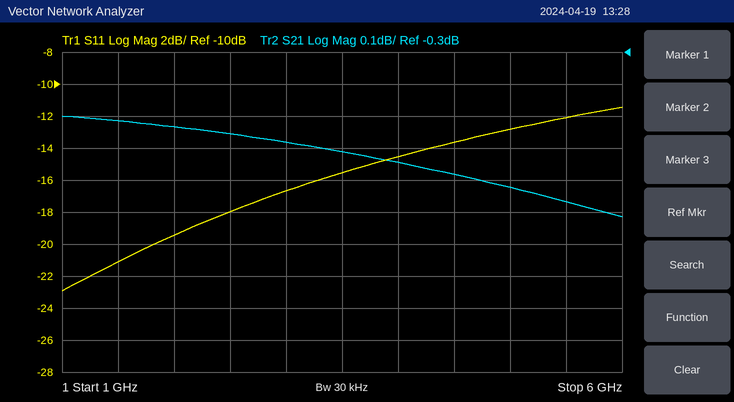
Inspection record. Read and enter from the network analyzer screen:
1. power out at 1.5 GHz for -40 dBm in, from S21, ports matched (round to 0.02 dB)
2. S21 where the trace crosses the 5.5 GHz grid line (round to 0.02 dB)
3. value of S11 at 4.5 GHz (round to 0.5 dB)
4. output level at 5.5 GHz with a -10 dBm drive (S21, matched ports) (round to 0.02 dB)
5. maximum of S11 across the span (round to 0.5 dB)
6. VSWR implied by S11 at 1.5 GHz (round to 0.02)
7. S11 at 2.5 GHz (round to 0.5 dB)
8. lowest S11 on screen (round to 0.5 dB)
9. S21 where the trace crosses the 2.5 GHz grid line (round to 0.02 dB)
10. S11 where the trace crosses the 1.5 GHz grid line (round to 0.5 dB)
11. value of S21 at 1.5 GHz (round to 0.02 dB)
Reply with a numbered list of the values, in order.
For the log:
1. -40.52 dBm
2. -0.76 dB
3. -13.5 dB
4. -10.76 dBm
5. -11.5 dB
6. 1.20
7. -18.0 dB
8. -23.0 dB
9. -0.56 dB
10. -21.0 dB
11. -0.52 dB
